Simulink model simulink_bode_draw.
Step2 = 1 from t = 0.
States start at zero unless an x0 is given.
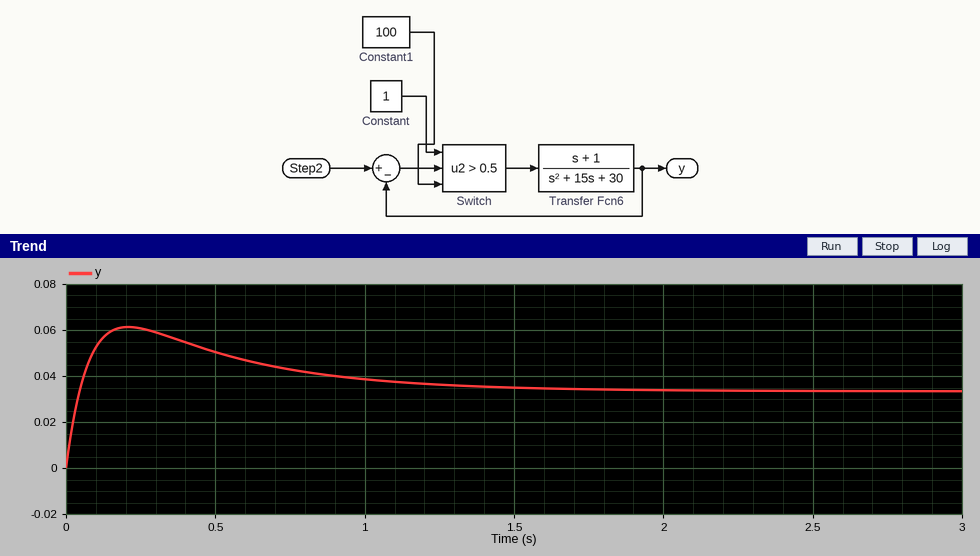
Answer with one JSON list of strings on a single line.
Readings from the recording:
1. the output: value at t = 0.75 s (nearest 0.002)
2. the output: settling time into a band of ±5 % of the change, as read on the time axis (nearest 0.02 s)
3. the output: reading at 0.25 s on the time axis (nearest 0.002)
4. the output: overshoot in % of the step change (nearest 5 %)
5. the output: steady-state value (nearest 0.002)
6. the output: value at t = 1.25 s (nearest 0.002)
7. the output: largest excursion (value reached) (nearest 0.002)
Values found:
["0.042", "1.48 s", "0.060", "85 %", "0.034", "0.036", "0.062"]
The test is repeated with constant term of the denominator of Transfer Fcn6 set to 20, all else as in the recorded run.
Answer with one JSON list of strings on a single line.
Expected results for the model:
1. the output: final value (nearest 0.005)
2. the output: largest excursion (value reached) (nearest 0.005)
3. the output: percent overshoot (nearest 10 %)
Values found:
["0.050", "0.065", "30 %"]
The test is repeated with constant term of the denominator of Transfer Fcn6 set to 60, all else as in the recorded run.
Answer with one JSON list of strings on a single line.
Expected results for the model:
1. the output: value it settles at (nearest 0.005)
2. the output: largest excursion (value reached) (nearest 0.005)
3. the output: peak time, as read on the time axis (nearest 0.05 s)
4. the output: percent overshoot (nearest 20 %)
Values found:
["0.015", "0.055", "0.15 s", "220 %"]
